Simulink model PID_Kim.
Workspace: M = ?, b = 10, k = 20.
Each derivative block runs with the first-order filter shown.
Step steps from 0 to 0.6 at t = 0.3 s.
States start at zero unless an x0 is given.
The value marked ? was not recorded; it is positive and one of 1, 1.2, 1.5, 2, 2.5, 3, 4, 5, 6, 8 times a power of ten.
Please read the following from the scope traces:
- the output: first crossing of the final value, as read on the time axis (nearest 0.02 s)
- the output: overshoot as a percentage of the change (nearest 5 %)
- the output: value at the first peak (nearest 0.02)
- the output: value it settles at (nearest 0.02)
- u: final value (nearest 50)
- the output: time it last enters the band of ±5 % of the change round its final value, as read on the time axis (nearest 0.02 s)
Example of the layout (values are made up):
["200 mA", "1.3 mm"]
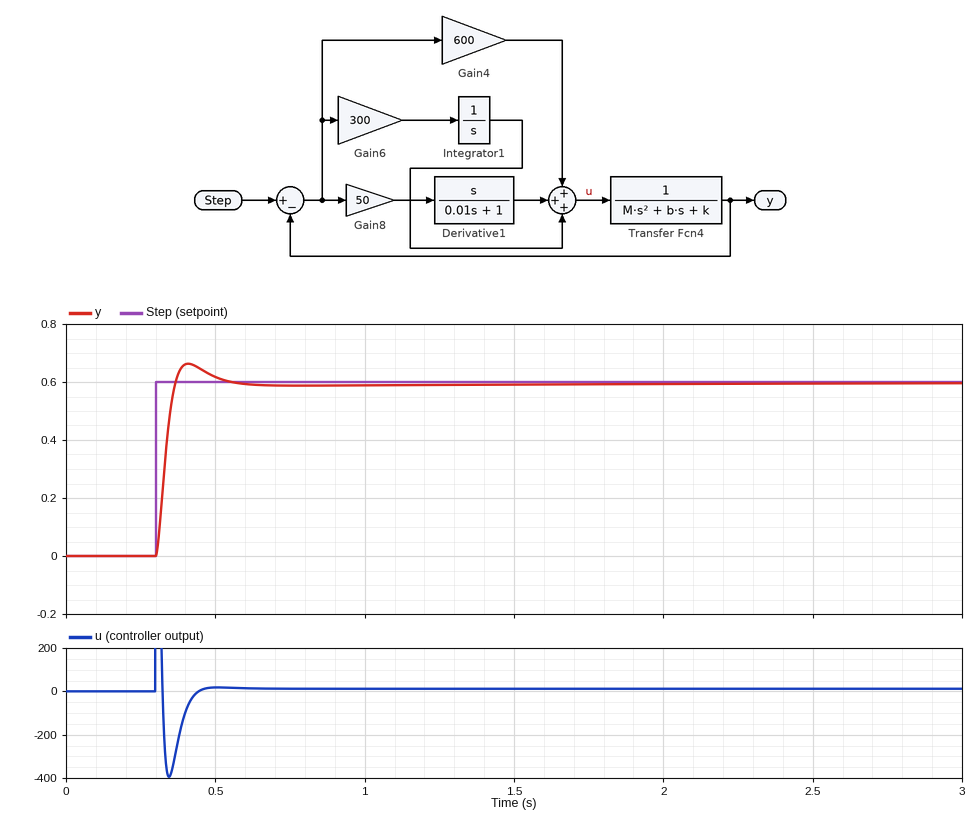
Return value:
["0.36 s", "10 %", "0.66", "0.60", "0", "0.48 s"]
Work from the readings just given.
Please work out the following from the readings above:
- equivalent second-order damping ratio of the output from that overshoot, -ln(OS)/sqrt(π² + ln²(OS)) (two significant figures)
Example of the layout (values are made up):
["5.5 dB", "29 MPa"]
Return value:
["0.59"]
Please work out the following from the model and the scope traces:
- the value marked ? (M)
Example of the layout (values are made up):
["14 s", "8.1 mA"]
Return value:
["2"]
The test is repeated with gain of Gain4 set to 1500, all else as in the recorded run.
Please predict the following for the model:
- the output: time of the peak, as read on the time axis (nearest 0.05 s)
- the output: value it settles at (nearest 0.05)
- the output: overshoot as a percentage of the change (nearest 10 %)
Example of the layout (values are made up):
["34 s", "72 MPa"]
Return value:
["0.40 s", "0.60", "30 %"]
